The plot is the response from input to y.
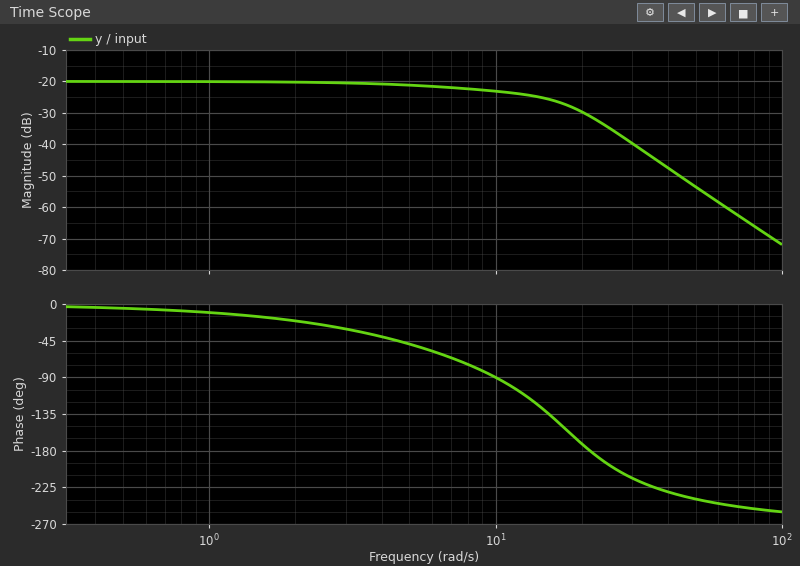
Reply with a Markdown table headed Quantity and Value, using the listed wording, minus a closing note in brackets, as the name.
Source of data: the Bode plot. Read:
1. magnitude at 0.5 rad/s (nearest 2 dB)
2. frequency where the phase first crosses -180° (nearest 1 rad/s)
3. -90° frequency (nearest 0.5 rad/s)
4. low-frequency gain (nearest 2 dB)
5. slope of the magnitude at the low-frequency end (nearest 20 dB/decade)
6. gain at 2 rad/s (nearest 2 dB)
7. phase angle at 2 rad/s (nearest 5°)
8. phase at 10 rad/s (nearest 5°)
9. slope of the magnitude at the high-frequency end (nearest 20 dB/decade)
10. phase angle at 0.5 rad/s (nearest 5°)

| Quantity | Value |
|---|---|
| magnitude at 0.5 rad/s | -20 dB |
| frequency where the phase first crosses -180° | 21 rad/s |
| -90° frequency | 10.0 rad/s |
| low-frequency gain | -20 dB |
| slope of the magnitude at the low-frequency end | 0 dB/decade |
| gain at 2 rad/s | -20 dB |
| phase angle at 2 rad/s | -20° |
| phase at 10 rad/s | -90° |
| slope of the magnitude at the high-frequency end | -60 dB/decade |
| phase angle at 0.5 rad/s | -5° |
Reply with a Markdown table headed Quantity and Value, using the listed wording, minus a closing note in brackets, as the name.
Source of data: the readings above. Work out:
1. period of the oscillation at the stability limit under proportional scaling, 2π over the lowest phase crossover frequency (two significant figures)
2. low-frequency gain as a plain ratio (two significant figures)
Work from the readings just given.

| Quantity | Value |
|---|---|
| period of the oscillation at the stability limit under proportional scaling, 2π over the lowest phase crossover frequency | 0.30 s |
| low-frequency gain as a plain ratio | 0.10 |
